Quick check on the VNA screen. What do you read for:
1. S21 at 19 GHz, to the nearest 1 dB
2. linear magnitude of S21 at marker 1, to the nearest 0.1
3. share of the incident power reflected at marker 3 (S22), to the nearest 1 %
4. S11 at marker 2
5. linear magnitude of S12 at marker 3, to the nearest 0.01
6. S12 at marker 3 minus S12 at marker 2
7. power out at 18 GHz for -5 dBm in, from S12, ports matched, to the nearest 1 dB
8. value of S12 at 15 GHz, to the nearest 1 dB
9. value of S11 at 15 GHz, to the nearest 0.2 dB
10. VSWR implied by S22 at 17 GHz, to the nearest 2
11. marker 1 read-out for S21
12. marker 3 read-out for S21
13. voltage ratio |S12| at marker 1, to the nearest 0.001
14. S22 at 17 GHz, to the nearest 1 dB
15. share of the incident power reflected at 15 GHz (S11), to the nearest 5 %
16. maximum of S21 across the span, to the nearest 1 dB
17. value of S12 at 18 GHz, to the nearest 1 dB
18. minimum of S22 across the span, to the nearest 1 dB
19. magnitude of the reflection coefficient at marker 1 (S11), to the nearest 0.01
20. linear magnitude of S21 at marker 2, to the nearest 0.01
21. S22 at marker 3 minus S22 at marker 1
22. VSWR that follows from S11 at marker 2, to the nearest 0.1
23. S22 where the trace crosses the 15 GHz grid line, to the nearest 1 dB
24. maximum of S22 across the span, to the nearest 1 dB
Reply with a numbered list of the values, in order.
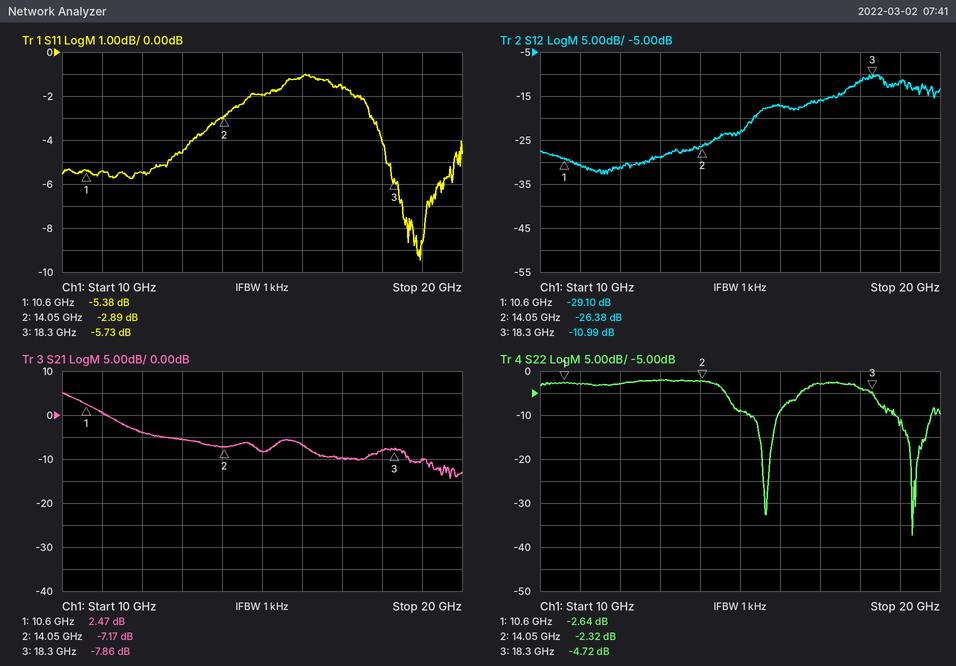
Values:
1. -10 dB
2. 1.3
3. 34 %
4. -2.89 dB
5. 0.28
6. 15.39 dB
7. -16 dBm
8. -23 dB
9. -2.0 dB
10. 6
11. 2.47 dB
12. -7.86 dB
13. 0.035
14. -3 dB
15. 65 %
16. 5 dB
17. -11 dB
18. -37 dB
19. 0.54
20. 0.44
21. -2.08 dB
22. 6.1
23. -9 dB
24. -2 dB
